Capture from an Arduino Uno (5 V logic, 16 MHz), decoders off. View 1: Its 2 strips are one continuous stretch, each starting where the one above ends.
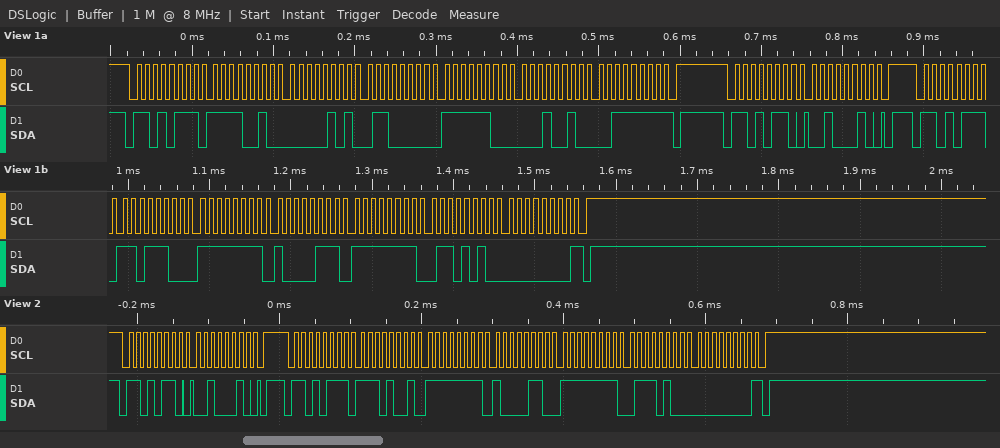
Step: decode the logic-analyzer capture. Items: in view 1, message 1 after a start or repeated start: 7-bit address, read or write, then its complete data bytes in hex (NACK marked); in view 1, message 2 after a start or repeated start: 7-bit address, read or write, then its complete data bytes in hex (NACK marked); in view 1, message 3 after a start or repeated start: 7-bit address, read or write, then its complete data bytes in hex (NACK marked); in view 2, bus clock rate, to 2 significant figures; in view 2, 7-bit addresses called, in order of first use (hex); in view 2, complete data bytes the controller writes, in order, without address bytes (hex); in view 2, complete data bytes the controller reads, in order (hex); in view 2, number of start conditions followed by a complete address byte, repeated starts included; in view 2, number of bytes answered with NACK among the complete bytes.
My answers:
0x6B read: F2 05 60 FC 12 3F NACK
0x6B write: 22
0x6B read: DC FF 87 FF 6A 00 NACK
100 kHz
0x6B
22
E9 FF 86 FF 74 00
2
1
